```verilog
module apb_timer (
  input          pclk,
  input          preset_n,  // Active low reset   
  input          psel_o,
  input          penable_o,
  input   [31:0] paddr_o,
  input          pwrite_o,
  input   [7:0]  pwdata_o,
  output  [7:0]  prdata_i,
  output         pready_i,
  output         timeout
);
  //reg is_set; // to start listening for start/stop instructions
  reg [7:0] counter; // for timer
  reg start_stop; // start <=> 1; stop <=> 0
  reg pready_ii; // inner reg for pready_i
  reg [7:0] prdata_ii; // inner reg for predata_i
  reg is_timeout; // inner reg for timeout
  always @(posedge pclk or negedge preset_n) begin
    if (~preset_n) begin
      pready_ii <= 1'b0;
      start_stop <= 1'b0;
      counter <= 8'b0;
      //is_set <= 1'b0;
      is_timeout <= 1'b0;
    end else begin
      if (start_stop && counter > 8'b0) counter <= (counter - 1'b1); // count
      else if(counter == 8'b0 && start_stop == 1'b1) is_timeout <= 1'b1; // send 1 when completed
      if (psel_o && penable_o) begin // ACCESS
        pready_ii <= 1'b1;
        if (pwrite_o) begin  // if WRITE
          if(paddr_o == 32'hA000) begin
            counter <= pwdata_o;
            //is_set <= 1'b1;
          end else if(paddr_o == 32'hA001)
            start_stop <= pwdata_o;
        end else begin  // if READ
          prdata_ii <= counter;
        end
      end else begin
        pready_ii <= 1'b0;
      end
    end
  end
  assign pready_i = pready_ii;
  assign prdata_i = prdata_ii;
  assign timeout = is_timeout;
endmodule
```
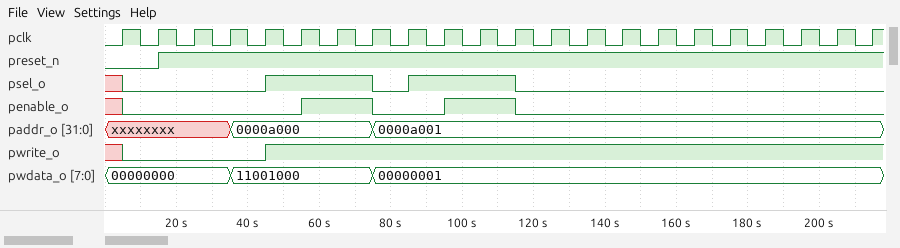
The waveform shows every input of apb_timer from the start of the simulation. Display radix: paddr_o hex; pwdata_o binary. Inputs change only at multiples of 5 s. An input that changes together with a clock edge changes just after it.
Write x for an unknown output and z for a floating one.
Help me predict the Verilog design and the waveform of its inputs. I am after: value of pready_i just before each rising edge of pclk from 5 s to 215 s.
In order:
0 0 0 0 0 0 0 1 1 0 0 1 1 0 0 0 0 0 0 0 0 0
